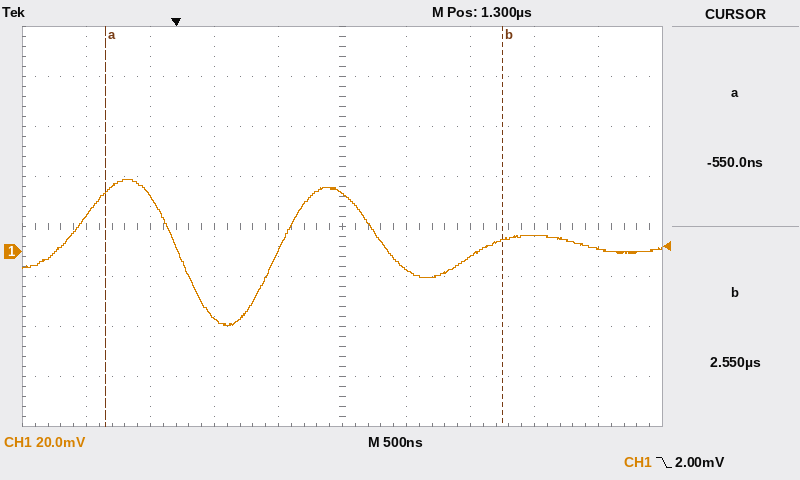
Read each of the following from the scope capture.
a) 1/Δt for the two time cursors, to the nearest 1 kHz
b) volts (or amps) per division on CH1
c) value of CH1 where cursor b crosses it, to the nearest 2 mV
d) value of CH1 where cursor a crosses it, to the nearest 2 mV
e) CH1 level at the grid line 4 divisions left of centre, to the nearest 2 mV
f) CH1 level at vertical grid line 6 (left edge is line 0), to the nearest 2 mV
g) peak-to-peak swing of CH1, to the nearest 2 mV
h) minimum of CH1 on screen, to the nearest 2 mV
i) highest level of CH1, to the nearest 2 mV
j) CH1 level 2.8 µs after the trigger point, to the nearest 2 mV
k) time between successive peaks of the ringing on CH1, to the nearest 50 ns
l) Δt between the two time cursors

323 kHz
20 mV
4 mV
24 mV
14 mV
-8 mV
58 mV
-30 mV
28 mV
6 mV
1.60 µs
3.10 µs
